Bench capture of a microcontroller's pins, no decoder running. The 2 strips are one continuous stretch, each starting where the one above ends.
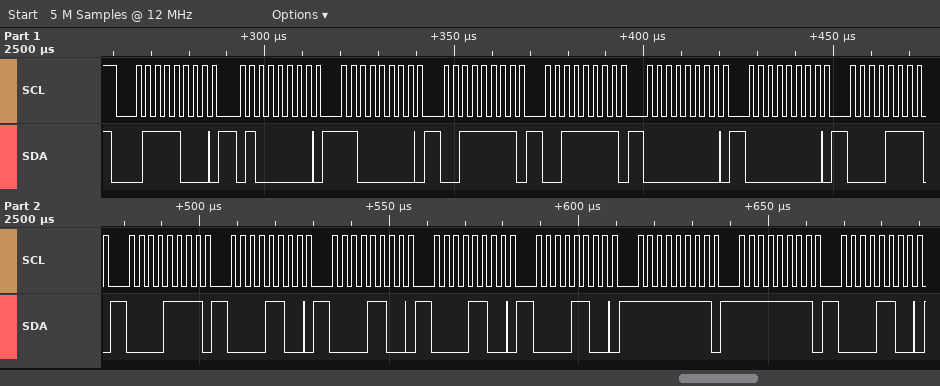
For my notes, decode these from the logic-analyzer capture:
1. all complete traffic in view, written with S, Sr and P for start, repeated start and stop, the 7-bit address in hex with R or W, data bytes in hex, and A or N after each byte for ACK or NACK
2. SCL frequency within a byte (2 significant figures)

S 3CW A 40 A C0 A 3F A 3F A 00 A 00 A 0F A 0F A 0C A 0C A 0C A 0C A FF A FF A 0C A
400 kHz
